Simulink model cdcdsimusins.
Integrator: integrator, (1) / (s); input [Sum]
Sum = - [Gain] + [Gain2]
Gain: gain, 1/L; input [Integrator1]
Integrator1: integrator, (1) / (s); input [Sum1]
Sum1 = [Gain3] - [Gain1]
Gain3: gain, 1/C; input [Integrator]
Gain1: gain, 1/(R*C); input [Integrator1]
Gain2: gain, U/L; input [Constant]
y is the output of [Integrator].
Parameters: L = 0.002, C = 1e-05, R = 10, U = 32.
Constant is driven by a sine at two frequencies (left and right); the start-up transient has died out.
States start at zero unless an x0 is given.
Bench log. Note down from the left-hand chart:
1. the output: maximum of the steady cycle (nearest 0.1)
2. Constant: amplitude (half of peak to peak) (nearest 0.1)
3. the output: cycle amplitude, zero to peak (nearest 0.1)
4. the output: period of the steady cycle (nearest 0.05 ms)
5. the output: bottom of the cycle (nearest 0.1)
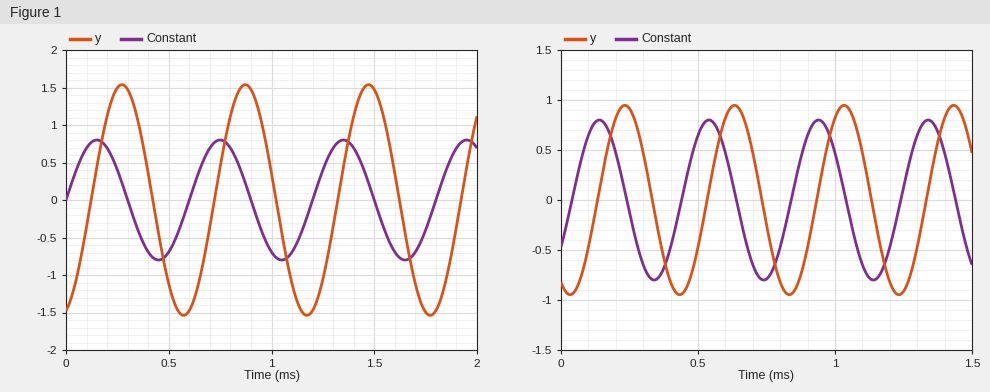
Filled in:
1.5
0.8
1.5
0.60 ms
-1.5
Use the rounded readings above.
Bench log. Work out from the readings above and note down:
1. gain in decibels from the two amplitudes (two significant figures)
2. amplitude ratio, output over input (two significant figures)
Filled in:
5.5 dB
1.9
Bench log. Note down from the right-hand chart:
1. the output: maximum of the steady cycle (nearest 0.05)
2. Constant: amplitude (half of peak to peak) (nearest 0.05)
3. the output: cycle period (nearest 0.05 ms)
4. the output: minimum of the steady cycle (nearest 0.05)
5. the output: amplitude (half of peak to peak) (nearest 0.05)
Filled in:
0.95
0.80
0.40 ms
-0.95
0.95
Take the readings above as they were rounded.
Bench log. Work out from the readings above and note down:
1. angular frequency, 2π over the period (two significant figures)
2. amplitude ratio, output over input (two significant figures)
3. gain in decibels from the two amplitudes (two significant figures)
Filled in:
16 rad/ms
1.2
1.5 dB
